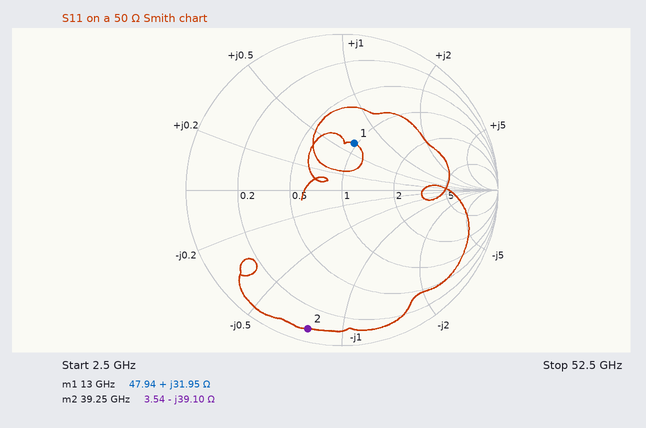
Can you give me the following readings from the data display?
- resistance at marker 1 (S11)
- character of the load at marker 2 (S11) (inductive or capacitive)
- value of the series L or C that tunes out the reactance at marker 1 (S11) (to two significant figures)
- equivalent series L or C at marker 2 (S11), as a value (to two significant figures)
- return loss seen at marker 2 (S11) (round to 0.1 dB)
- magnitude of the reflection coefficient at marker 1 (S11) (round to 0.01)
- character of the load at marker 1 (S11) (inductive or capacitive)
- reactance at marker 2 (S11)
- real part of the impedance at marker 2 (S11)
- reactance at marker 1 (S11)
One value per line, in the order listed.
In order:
47.94 Ω
capacitive
380 fF
100 fF
0.8 dB
0.31
inductive
-39.10 Ω
3.54 Ω
+31.95 Ω
